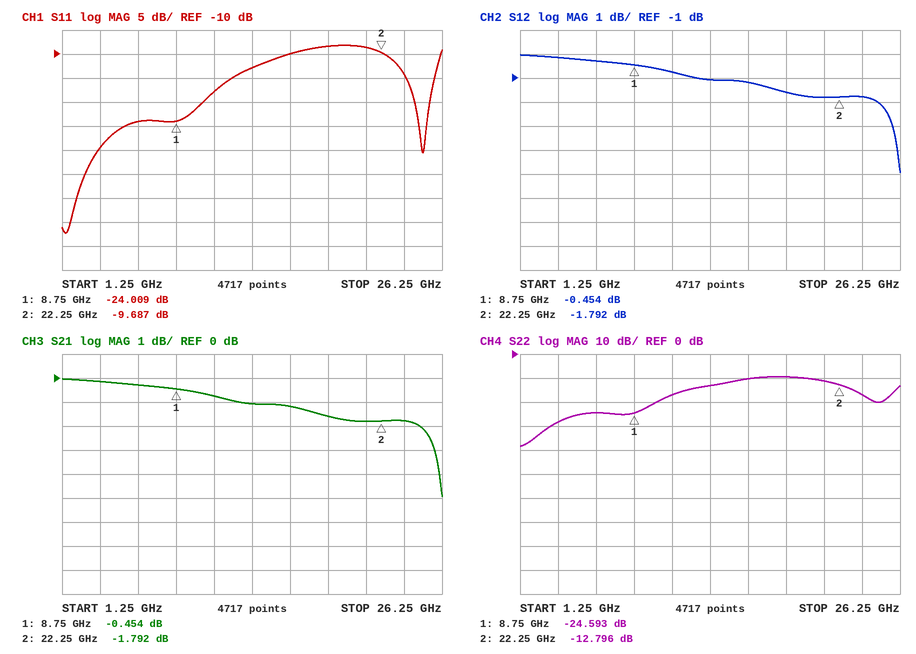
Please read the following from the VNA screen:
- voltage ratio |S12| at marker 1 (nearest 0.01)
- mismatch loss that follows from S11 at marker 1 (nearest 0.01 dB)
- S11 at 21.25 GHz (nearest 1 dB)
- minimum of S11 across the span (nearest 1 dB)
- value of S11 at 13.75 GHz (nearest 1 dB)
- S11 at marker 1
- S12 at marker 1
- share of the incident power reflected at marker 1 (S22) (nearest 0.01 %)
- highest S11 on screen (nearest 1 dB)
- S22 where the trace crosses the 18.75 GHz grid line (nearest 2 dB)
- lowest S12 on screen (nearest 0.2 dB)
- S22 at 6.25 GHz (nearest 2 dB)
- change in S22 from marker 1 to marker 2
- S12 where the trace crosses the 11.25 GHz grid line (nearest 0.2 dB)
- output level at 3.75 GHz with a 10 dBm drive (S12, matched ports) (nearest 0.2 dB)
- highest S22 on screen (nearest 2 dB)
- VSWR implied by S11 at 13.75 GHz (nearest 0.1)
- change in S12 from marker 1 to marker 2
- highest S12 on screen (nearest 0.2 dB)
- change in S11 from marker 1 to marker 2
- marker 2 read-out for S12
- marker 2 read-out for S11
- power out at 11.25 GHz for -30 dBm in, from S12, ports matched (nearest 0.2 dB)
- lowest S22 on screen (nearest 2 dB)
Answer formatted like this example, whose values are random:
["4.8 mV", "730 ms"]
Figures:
["0.95", "0.02 dB", "-9 dB", "-47 dB", "-13 dB", "-24.009 dB", "-0.454 dB", "0.35 %", "-8 dB", "-10 dB", "-5.0 dB", "-24 dB", "11.797 dB", "-0.8 dB", "9.8 dBm", "-10 dB", "1.6", "-1.338 dB", "0.0 dB", "14.322 dB", "-1.792 dB", "-9.687 dB", "-30.8 dBm", "-38 dB"]
